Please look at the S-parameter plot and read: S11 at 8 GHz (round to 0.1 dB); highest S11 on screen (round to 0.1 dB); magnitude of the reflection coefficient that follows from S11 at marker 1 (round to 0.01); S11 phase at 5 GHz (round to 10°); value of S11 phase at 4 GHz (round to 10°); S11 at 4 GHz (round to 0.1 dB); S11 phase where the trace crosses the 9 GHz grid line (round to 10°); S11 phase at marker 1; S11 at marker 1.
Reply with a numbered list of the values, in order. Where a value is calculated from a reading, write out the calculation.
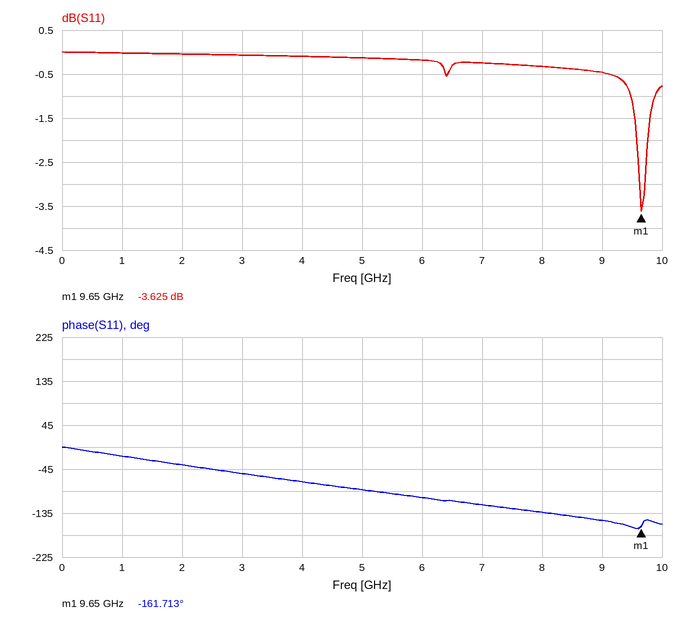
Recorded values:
1. -0.3 dB
2. 0.0 dB
3. 10^(-3.625/20) ≈ 0.66
4. -90°
5. -70°
6. -0.1 dB
7. -150°
8. -161.713°
9. -3.625 dB
